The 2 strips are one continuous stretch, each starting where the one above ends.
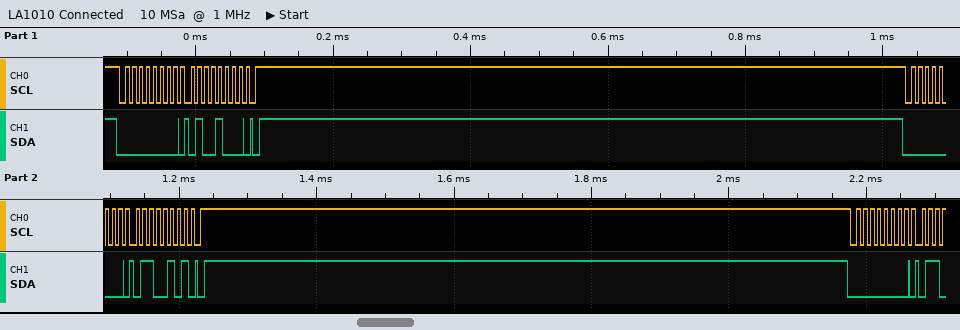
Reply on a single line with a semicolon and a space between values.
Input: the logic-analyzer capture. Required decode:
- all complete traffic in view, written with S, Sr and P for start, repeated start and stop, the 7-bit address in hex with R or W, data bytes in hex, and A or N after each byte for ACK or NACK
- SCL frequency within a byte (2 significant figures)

S 00W A 48 A P S 00W A 65 A P S 00W A; 100 kHz
